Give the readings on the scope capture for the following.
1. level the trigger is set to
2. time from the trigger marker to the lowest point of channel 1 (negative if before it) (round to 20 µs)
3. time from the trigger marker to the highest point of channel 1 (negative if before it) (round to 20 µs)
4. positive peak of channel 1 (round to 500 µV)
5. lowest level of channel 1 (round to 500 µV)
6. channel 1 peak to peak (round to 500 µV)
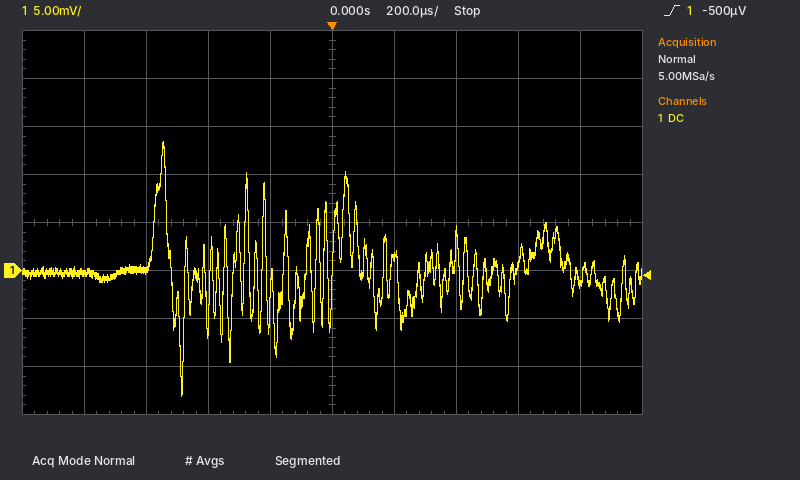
-500 µV
-480 µs
-540 µs
13.5 mV
-13.0 mV
26.5 mV
